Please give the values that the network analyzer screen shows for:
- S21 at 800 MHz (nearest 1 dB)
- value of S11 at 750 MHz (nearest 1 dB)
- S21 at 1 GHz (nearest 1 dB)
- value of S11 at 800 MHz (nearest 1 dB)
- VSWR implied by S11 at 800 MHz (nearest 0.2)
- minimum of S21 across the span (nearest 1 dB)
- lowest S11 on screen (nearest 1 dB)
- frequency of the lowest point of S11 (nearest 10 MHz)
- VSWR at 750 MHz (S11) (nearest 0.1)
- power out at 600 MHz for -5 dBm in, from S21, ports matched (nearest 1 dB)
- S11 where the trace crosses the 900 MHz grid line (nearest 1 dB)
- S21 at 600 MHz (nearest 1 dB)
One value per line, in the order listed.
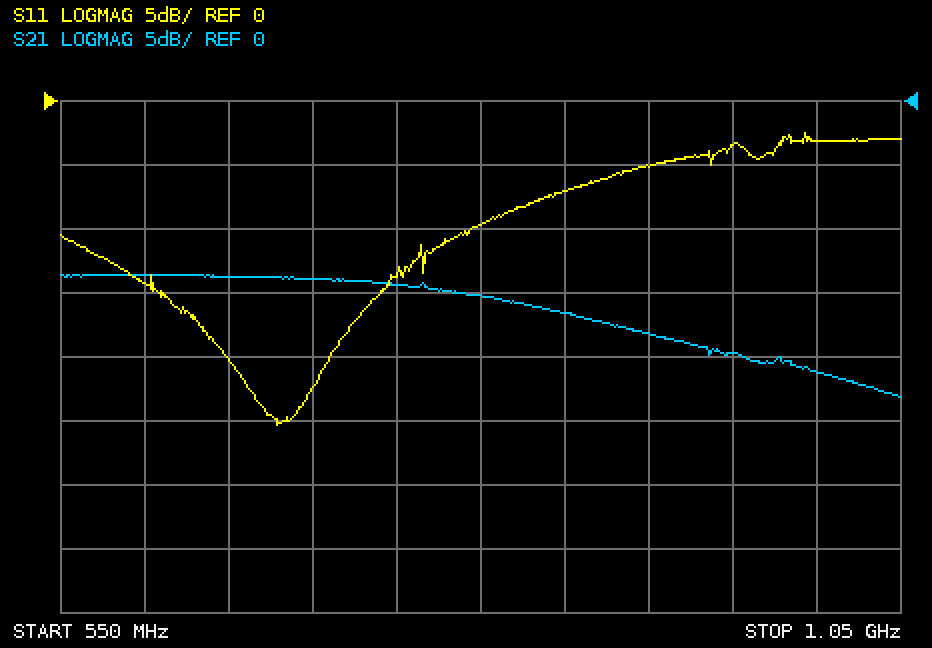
-15 dB
-14 dB
-21 dB
-10 dB
2.0
-23 dB
-25 dB
680 MHz
1.5
-19 dBm
-5 dB
-14 dB
